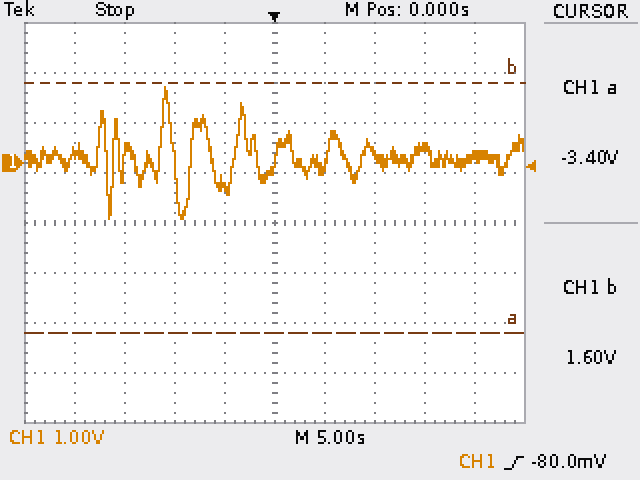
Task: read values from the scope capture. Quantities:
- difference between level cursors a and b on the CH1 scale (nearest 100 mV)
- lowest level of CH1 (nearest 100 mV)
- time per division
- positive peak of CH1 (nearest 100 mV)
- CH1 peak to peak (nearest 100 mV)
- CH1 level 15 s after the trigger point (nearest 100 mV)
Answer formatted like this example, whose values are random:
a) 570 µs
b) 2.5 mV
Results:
a) 5.0 V
b) -1.1 V
c) 5 s
d) 1.5 V
e) 2.6 V
f) 300 mV
